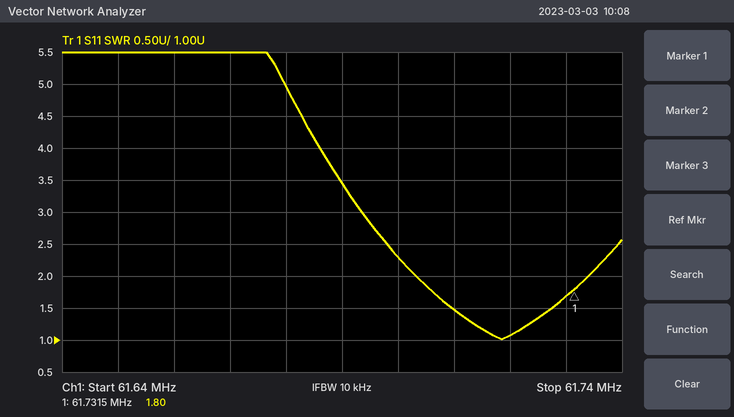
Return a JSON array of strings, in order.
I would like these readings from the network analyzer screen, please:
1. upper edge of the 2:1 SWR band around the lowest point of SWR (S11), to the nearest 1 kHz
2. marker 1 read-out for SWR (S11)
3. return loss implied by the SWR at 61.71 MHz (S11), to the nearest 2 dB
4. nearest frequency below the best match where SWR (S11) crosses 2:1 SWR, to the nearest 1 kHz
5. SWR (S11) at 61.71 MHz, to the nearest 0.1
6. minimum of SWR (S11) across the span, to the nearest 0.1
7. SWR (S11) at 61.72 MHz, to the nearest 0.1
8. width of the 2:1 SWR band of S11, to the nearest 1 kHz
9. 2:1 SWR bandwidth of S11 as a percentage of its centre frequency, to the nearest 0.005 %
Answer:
["61.734 MHz", "1.80", "14 dB", "61.703 MHz", "1.5", "1.0", "1.1", "31 kHz", "0.050 %"]
